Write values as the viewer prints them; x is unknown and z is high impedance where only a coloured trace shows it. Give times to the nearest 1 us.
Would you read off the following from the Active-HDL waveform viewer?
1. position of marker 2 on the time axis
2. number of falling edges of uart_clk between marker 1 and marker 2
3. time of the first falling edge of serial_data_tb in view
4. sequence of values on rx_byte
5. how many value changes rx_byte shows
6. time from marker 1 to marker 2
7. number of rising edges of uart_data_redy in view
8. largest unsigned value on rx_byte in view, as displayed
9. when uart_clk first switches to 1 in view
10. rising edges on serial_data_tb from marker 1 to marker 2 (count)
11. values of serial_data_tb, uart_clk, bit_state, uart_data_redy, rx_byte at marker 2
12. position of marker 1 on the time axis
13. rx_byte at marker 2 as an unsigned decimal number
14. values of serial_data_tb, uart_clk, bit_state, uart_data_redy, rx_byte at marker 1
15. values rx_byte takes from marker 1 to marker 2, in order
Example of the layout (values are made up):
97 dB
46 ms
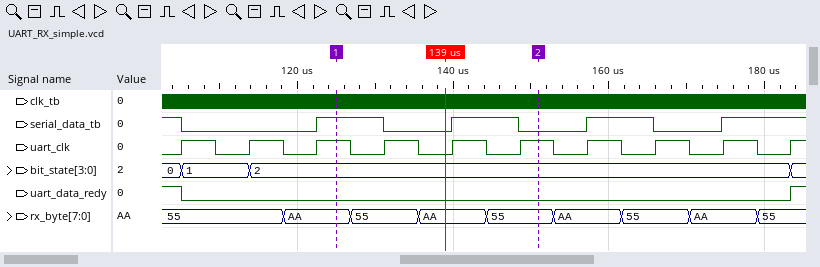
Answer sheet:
151 us
3
105 us
55, AA, 55, AA, 55, AA, 55, AA, 55
8
26 us
1
AA
105 us
1
serial_data_tb=0, uart_clk=1, bit_state=2, uart_data_redy=0, rx_byte=55
125 us
85
serial_data_tb=1, uart_clk=1, bit_state=2, uart_data_redy=0, rx_byte=AA
AA, 55, AA, 55
